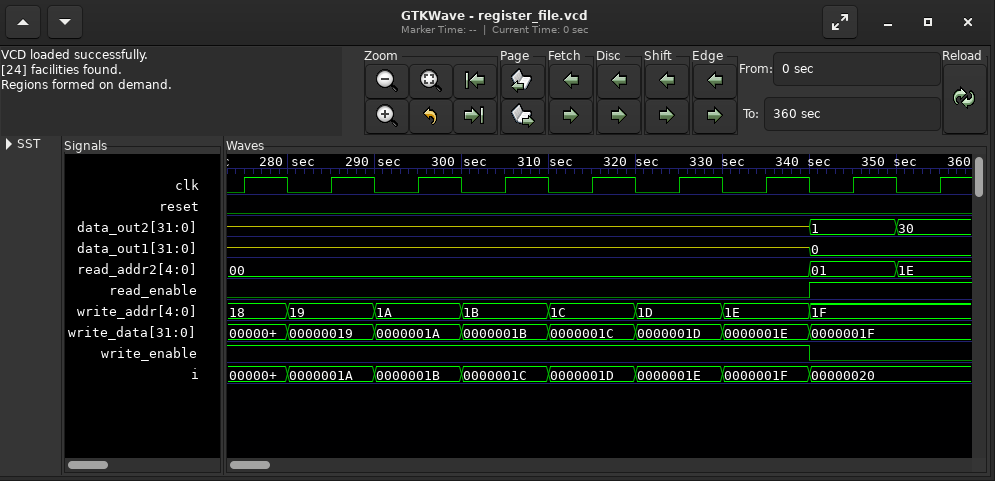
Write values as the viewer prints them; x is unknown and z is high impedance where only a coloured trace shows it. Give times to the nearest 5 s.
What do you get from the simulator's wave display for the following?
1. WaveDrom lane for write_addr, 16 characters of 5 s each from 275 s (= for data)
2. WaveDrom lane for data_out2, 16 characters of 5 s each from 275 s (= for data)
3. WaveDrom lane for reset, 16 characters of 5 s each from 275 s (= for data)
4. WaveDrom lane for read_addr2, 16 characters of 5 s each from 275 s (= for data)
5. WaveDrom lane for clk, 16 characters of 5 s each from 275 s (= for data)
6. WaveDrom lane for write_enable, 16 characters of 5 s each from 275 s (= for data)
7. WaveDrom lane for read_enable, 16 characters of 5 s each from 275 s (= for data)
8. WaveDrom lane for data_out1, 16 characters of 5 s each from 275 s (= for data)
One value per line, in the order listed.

{name: 'write_addr', wave: '==.=.=.=.=.=.=..', data: '18 19 1A 1B 1C 1D 1E 1F'}
{name: 'data_out2', wave: 'z............=.=', data: '1 30'}
{name: 'reset', wave: '0...............'}
{name: 'read_addr2', wave: '=............=.=', data: '00 01 1E'}
{name: 'clk', wave: '1010101010101010'}
{name: 'write_enable', wave: '1............0..'}
{name: 'read_enable', wave: '0............1..'}
{name: 'data_out1', wave: 'z............=..', data: '0'}
